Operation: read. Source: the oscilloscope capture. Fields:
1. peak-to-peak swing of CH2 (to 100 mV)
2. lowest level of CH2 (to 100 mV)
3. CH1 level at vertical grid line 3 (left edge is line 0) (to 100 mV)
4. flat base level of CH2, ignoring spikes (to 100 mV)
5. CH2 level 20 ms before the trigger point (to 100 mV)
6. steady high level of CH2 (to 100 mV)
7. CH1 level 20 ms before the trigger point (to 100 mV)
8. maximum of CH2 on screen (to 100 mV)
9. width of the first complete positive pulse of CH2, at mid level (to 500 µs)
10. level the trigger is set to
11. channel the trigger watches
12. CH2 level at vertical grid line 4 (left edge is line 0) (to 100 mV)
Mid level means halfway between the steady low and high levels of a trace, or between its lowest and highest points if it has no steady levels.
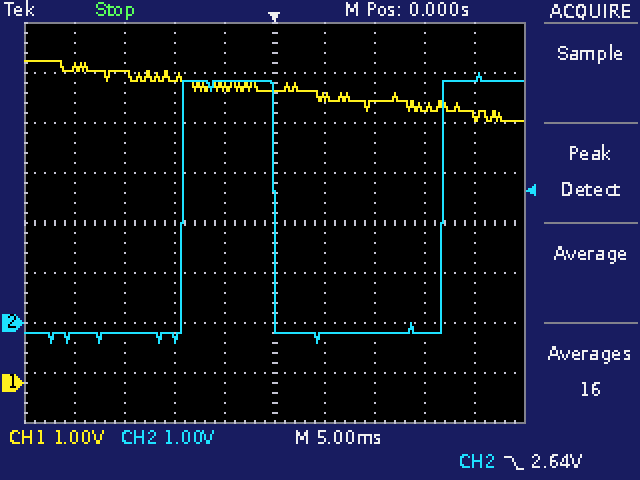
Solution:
5.4 V
-400 mV
6.1 V
-200 mV
-200 mV
4.8 V
6.3 V
5.0 V
9.0 ms
2.64 V
CH2
4.8 V
